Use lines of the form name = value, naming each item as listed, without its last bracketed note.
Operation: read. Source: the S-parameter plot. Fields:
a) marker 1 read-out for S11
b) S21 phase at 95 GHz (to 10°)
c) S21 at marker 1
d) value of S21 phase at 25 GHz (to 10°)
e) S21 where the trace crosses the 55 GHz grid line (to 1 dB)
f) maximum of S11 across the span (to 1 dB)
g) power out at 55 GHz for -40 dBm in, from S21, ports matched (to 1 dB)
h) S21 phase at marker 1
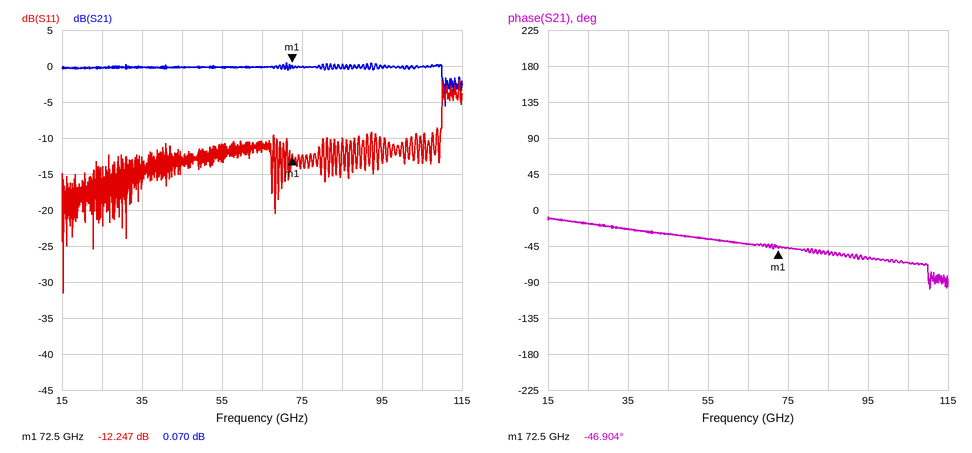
marker 1 read-out for S11 = -12.247 dB
S21 phase at 95 GHz = -60°
S21 at marker 1 = 0.070 dB
value of S21 phase at 25 GHz = -20°
S21 where the trace crosses the 55 GHz grid line = 0 dB
maximum of S11 across the span = -2 dB
power out at 55 GHz for -40 dBm in, from S21, ports matched = -40 dBm
S21 phase at marker 1 = -46.904°
